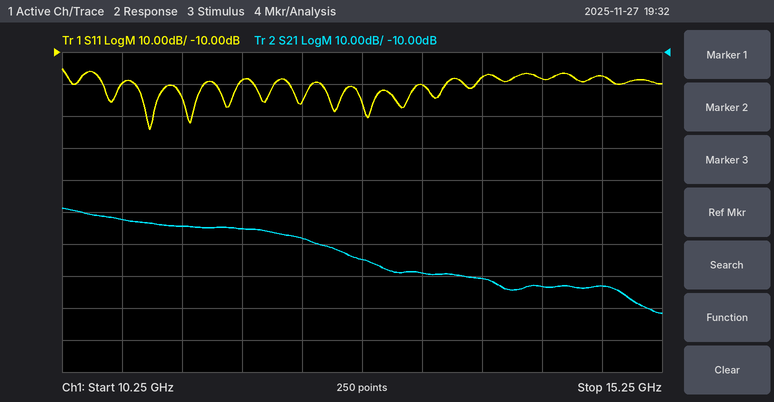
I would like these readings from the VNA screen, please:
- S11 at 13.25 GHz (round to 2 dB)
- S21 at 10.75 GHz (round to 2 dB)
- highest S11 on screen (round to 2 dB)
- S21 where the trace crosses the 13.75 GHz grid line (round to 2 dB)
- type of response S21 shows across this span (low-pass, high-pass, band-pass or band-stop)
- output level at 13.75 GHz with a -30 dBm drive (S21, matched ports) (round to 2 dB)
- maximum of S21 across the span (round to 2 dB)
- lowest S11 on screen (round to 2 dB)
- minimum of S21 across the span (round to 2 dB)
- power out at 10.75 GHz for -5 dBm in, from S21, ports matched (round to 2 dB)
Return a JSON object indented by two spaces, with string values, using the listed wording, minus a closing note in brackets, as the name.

{
  "S11 at 13.25 GHz": "-20 dB",
  "S21 at 10.75 GHz": "-62 dB",
  "highest S11 on screen": "-16 dB",
  "S21 where the trace crosses the 13.75 GHz grid line": "-80 dB",
  "type of response S21 shows across this span": "low-pass",
  "output level at 13.75 GHz with a -30 dBm drive (S21, matched ports)": "-110 dBm",
  "maximum of S21 across the span": "-58 dB",
  "lowest S11 on screen": "-34 dB",
  "minimum of S21 across the span": "-92 dB",
  "power out at 10.75 GHz for -5 dBm in, from S21, ports matched": "-68 dBm"
}
